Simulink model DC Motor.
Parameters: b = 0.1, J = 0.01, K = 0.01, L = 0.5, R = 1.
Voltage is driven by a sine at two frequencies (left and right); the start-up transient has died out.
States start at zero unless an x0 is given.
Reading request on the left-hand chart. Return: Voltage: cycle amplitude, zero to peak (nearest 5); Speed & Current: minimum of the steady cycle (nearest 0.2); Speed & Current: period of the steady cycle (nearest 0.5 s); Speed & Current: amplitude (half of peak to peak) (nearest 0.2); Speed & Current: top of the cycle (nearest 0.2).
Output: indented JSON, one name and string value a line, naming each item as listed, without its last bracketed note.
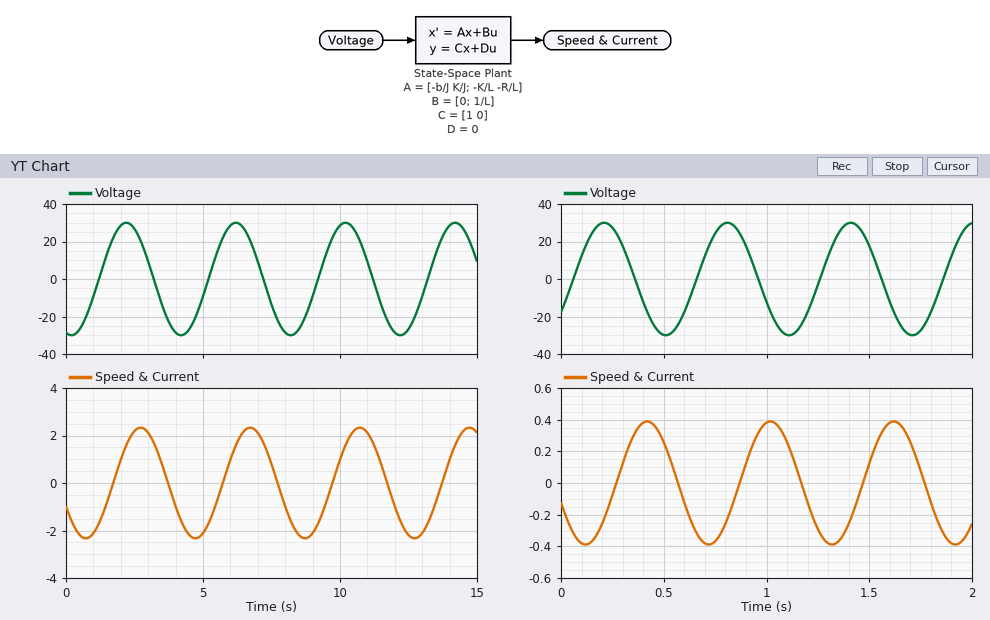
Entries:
{
  "Voltage: cycle amplitude, zero to peak": "30",
  "Speed & Current: minimum of the steady cycle": "-2.4",
  "Speed & Current: period of the steady cycle": "4.0 s",
  "Speed & Current: amplitude (half of peak to peak)": "2.4",
  "Speed & Current: top of the cycle": "2.4"
}
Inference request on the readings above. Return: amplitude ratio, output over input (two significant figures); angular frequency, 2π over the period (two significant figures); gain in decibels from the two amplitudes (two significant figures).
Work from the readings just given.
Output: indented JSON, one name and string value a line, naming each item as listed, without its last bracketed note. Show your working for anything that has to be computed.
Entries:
{
  "amplitude ratio, output over input": "2.4 / 30 = 0.080",
  "angular frequency, 2π over the period": "2π / 4 = 1.6 rad/s",
  "gain in decibels from the two amplitudes": "20 log10(2.4 / 30) = -22 dB"
}
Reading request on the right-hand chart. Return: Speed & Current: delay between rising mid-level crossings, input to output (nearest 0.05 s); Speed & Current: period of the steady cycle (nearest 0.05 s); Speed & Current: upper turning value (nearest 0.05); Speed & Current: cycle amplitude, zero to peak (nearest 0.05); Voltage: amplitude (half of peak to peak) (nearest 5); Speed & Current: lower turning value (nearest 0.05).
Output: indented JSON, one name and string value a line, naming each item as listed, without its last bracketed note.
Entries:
{
  "Speed & Current: delay between rising mid-level crossings, input to output": "0.20 s",
  "Speed & Current: period of the steady cycle": "0.60 s",
  "Speed & Current: upper turning value": "0.40",
  "Speed & Current: cycle amplitude, zero to peak": "0.40",
  "Voltage: amplitude (half of peak to peak)": "30",
  "Speed & Current: lower turning value": "-0.40"
}
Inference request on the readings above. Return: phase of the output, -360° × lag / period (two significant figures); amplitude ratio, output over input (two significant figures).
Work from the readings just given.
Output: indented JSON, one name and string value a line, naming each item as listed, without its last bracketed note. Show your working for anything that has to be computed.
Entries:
{
  "phase of the output, -360° × lag / period": "-360 × 0.2 / 0.6 = -120°",
  "amplitude ratio, output over input": "0.4 / 30 = 0.013"
}
